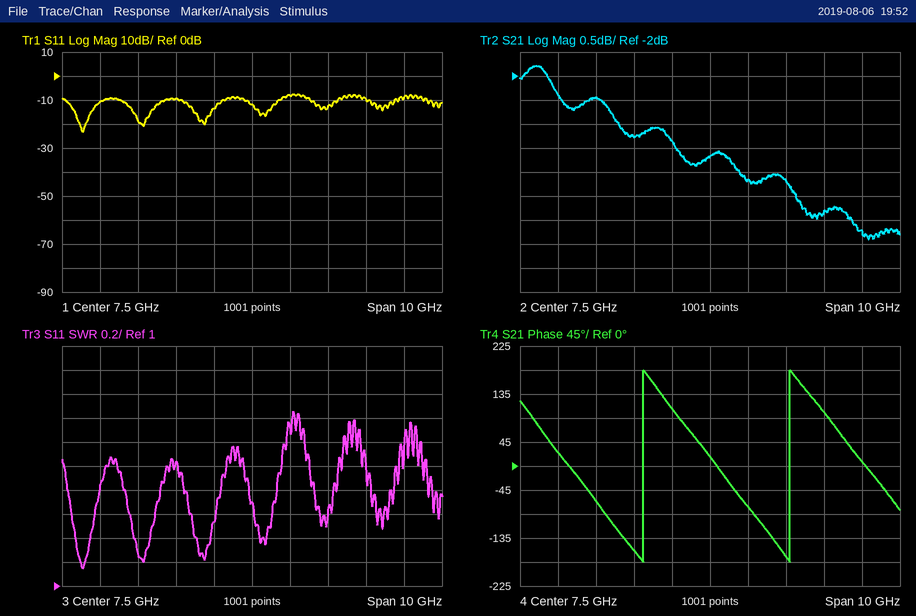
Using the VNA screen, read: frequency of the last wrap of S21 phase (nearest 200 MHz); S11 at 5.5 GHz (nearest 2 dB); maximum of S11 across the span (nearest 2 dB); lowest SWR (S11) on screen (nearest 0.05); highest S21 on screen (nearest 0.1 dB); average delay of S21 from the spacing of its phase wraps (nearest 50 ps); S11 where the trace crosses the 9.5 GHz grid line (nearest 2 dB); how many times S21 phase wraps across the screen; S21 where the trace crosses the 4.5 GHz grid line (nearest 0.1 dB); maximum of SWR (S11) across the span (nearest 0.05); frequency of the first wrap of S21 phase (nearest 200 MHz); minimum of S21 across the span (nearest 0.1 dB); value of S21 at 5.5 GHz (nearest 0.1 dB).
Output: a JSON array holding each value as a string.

["9.6 GHz", "-10 dB", "-8 dB", "1.15", "-1.8 dB", "250 ps", "-12 dB", "2", "-2.5 dB", "2.45", "5.8 GHz", "-5.4 dB", "-3.3 dB"]
